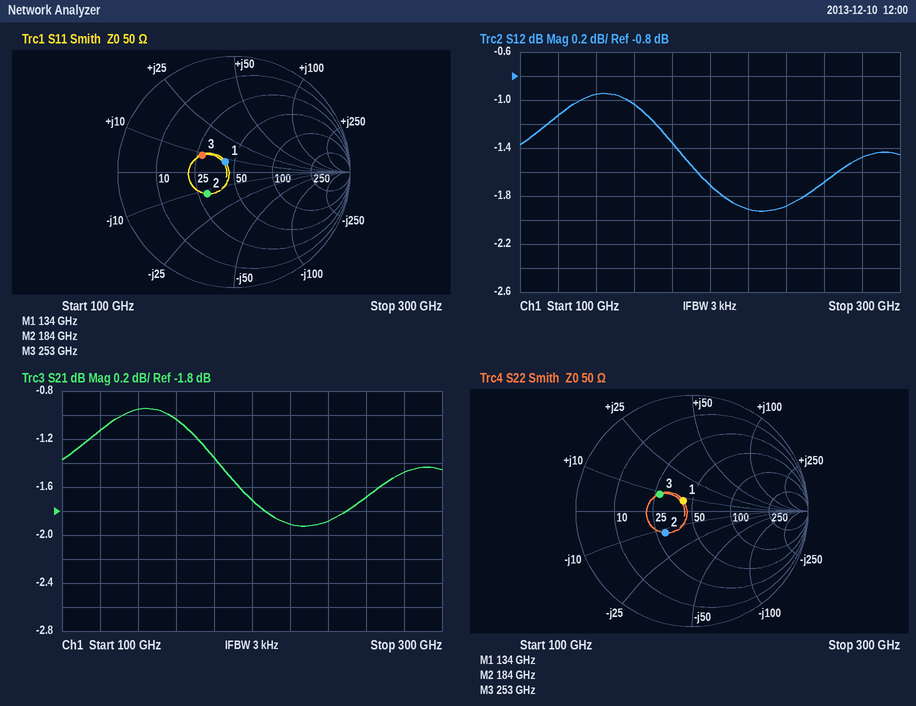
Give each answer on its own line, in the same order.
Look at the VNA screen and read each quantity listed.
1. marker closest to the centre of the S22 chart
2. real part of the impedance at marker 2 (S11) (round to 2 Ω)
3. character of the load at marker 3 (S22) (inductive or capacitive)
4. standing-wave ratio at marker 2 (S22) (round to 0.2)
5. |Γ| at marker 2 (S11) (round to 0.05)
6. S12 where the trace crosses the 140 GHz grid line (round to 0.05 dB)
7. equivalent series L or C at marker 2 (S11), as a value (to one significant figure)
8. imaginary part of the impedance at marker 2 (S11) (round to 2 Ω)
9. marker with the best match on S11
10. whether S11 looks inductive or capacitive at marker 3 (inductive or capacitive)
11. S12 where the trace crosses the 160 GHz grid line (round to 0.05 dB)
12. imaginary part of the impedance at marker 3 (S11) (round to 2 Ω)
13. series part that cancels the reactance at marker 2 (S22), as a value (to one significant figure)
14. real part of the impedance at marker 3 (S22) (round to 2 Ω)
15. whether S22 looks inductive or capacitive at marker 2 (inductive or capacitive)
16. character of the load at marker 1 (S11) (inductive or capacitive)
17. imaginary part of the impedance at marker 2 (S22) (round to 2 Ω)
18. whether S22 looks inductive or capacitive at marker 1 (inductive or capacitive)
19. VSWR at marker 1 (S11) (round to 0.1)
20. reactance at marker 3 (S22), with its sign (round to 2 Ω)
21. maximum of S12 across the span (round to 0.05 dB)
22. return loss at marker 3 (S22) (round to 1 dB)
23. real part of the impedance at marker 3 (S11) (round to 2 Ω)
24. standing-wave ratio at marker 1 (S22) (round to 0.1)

marker 1
30 Ω
inductive
1.8
0.30
-0.95 dB
70 fF
-12 Ω
marker 1
inductive
-1.05 dB
+8 Ω
10 pH
28 Ω
capacitive
inductive
-12 Ω
inductive
1.3
+8 Ω
-0.95 dB
10 dB
28 Ω
1.3
